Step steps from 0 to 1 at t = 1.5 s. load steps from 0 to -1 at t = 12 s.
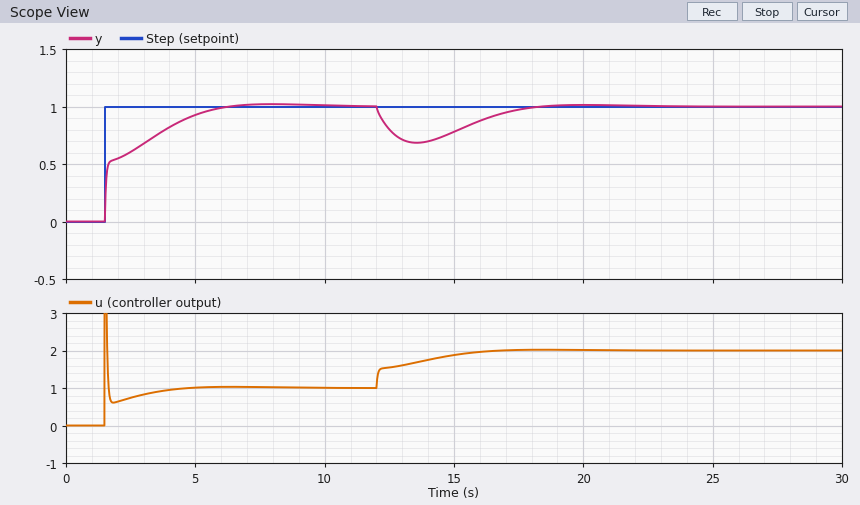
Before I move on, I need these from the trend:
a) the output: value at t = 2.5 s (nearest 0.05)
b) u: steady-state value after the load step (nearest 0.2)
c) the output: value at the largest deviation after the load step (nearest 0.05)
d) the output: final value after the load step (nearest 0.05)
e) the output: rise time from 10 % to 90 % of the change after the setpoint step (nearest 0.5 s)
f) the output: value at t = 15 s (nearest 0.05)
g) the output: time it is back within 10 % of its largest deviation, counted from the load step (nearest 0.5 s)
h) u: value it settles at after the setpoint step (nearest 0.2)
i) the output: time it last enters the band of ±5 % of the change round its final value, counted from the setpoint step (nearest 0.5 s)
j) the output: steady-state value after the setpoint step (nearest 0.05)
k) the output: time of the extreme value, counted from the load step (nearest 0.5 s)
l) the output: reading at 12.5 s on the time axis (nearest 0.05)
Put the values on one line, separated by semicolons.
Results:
0.60; 2.0; 0.70; 1.00; 3.0 s; 0.80; 5.5 s; 1.0; 4.0 s; 1.00; 1.5 s; 0.80
